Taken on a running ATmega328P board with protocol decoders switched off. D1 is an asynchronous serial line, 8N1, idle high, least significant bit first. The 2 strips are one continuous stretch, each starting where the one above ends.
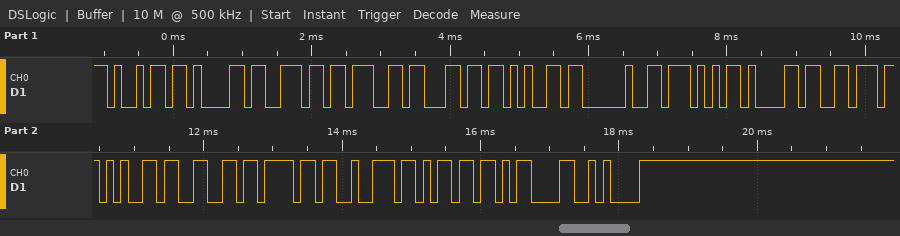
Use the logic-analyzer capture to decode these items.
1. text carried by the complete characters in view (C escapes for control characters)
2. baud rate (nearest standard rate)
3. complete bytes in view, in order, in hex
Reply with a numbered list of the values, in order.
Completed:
1. "iangle Waveform\r\n"
2. 9600 baud
3. 0x69 0x61 0x6E 0x67 0x6C 0x65 0x20 0x57 0x61 0x76 0x65 0x66 0x6F 0x72 0x6D 0x0D 0x0A
